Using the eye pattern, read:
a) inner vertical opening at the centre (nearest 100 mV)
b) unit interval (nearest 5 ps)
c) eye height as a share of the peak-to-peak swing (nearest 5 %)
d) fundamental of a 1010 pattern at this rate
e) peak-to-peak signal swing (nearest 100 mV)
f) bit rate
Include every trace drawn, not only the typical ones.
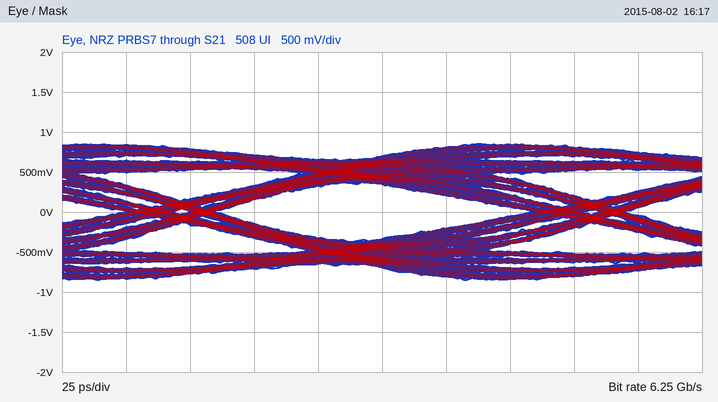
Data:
700 mV
160 ps
40 %
3.125 GHz
1.7 V
6.25 Gb/s
